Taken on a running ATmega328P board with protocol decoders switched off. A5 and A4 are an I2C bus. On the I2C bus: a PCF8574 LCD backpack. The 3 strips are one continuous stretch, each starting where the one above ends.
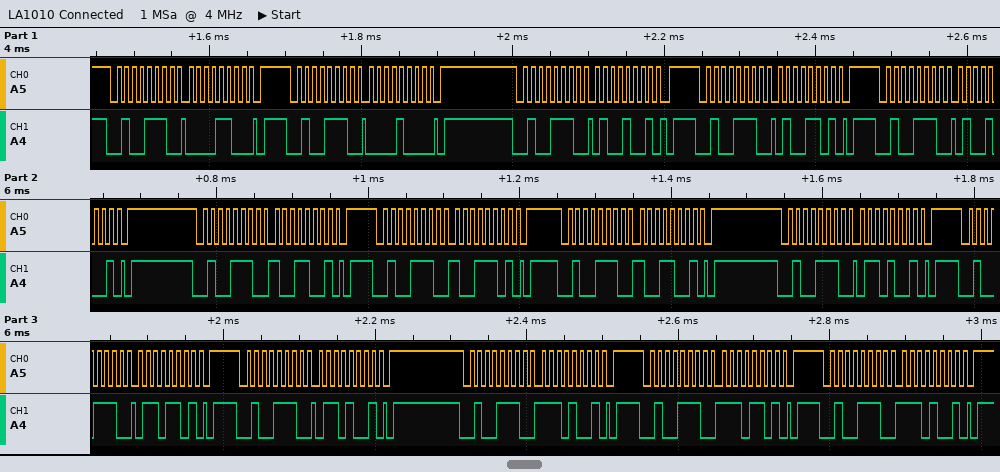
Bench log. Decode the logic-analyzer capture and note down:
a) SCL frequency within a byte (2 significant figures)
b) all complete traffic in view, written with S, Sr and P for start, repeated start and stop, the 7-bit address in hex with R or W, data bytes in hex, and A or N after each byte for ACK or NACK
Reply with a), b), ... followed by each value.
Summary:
a) 100 kHz
b) S 27W A 0C A P S 27W A 08 A P S 27W A 49 A P S 27W A 4D A P S 27W A 49 A P S 27W A 99 A P S 27W A 9D A P S 27W A 99 A P S 27W A 69 A P S 27W A 6D A P S 27W A 69 A P S 27W A E9 A P S 27W A ED A P S 27W A E9 A P
